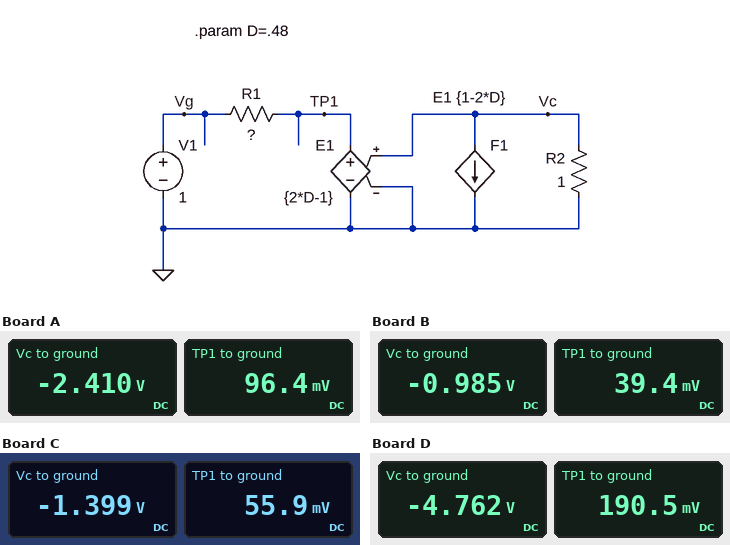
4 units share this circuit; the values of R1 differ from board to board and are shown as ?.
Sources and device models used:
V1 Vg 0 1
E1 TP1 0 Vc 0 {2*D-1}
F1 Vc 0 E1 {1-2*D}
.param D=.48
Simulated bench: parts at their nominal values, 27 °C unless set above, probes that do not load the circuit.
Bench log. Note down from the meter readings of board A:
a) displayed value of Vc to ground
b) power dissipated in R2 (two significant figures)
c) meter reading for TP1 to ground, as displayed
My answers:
-2.410 V
5.8 W
96.4 mV
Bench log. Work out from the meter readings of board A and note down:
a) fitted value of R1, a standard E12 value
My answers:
0.015 Ω
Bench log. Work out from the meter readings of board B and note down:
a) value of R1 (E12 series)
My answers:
0.039 Ω
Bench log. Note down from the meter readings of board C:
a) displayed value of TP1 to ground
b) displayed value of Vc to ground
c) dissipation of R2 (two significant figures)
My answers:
55.9 mV
-1.399 V
2.0 W
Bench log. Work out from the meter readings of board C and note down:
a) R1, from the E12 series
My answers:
0.027 Ω
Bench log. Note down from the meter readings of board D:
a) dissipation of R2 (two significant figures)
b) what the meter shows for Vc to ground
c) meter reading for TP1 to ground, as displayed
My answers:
23 W
-4.762 V
190.5 mV
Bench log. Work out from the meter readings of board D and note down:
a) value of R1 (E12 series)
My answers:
6.8 mΩ
